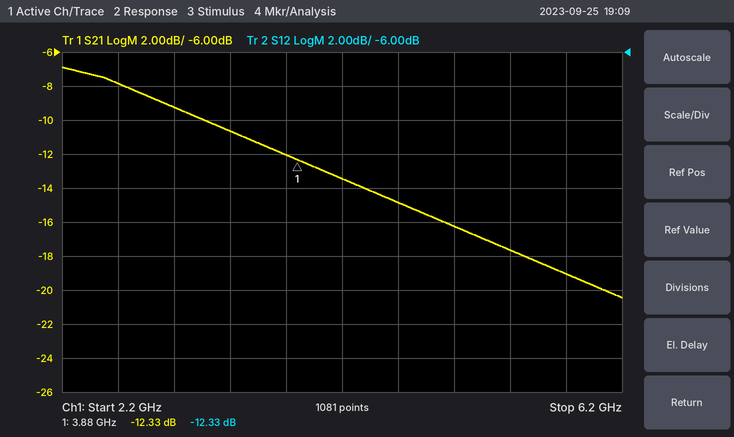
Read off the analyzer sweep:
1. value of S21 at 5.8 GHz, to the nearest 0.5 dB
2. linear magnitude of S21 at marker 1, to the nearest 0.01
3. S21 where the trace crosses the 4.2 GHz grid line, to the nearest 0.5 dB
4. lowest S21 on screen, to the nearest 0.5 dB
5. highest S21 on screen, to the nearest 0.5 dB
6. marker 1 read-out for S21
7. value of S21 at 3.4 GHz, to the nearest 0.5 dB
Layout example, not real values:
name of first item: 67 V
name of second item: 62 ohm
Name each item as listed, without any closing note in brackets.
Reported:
value of S21 at 5.8 GHz, to the nearest 0.5 dB: -19.0 dB
linear magnitude of S21 at marker 1, to the nearest 0.01: 0.24
S21 where the trace crosses the 4.2 GHz grid line, to the nearest 0.5 dB: -13.5 dB
lowest S21 on screen, to the nearest 0.5 dB: -20.5 dB
highest S21 on screen, to the nearest 0.5 dB: -7.0 dB
marker 1 read-out for S21: -12.33 dB
value of S21 at 3.4 GHz, to the nearest 0.5 dB: -10.5 dB
